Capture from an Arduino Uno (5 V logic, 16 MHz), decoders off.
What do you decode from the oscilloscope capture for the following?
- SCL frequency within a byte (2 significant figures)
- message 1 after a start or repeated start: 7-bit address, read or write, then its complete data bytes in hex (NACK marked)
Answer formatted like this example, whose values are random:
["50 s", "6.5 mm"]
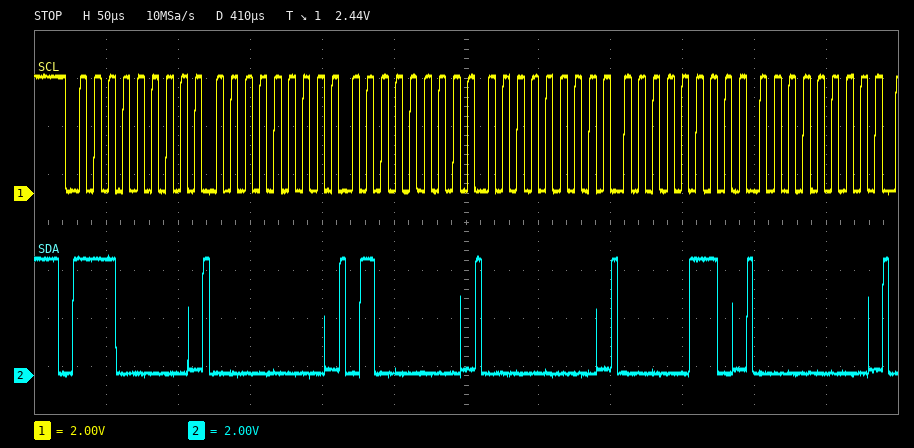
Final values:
["100 kHz", "0x70 write: 00 40 00 06 00"]
